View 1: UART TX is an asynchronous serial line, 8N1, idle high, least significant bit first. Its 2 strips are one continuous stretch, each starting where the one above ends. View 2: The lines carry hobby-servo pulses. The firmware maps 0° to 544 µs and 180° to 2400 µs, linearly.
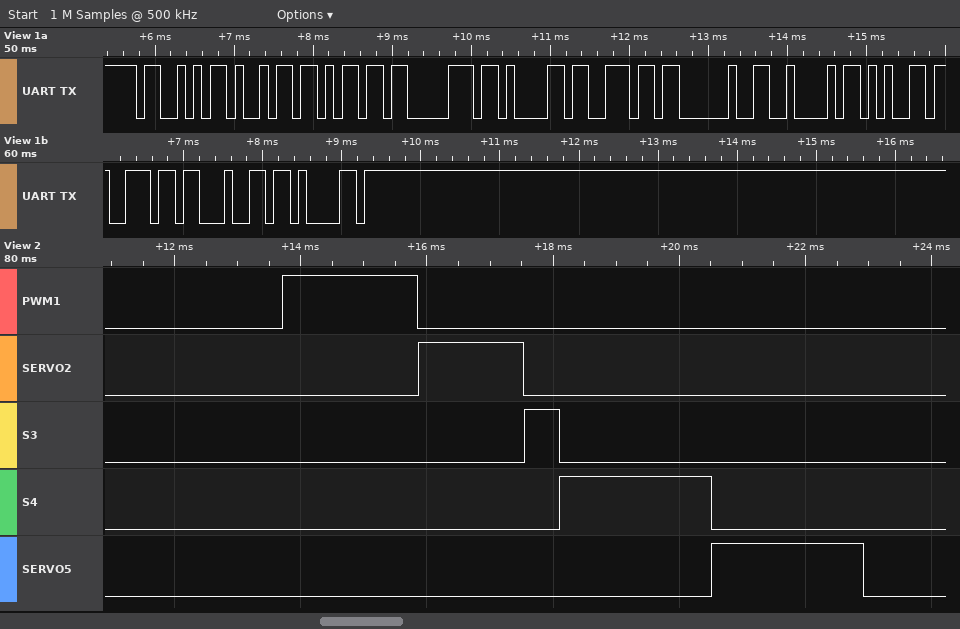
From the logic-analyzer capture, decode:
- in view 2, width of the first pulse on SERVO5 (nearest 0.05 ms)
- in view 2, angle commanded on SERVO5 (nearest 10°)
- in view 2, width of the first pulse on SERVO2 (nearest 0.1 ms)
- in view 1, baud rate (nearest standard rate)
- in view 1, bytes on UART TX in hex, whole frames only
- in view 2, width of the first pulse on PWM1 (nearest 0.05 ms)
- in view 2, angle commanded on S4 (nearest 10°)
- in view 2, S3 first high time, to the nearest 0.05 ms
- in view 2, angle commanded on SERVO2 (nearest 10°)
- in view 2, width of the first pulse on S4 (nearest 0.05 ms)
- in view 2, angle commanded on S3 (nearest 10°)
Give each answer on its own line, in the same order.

2.40 ms
180°
1.7 ms
9600 baud
53 69 6D 70 61 6E 20 42 65 6E 64 61
2.15 ms
180°
0.55 ms
110°
2.40 ms
0°
